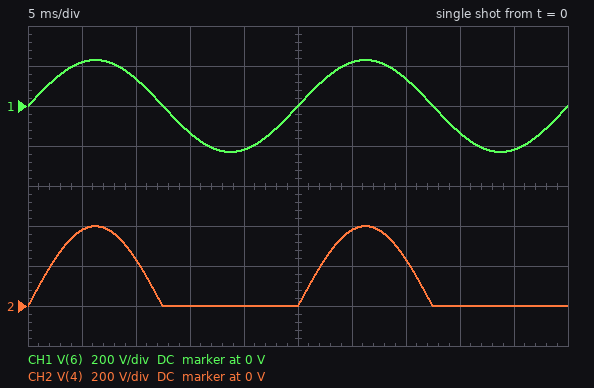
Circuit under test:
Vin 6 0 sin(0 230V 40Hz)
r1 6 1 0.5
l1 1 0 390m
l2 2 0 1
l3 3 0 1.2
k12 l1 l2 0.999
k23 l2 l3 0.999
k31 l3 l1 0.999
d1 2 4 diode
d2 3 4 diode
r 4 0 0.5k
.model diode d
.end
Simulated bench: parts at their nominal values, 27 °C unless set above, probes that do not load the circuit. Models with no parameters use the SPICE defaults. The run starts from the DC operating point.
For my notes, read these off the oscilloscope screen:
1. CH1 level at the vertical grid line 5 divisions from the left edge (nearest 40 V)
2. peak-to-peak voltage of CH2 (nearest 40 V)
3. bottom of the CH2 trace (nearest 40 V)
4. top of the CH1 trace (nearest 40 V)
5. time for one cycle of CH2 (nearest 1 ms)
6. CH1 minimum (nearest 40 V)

0 V
400 V
0 V
240 V
25 ms
-240 V
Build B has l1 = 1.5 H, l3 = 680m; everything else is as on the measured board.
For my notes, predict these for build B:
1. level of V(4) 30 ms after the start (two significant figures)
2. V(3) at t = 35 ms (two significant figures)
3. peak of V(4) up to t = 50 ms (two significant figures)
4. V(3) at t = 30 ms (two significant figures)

180 V
91 V
190 V
150 V
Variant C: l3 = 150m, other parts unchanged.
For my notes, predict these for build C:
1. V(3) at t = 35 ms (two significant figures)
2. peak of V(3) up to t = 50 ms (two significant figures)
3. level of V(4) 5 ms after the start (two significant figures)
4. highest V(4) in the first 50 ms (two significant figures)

82 V
140 V
350 V
360 V
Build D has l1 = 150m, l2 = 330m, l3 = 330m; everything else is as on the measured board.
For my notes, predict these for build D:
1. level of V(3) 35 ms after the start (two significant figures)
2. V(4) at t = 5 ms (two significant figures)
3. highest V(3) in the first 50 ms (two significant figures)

190 V
320 V
340 V
